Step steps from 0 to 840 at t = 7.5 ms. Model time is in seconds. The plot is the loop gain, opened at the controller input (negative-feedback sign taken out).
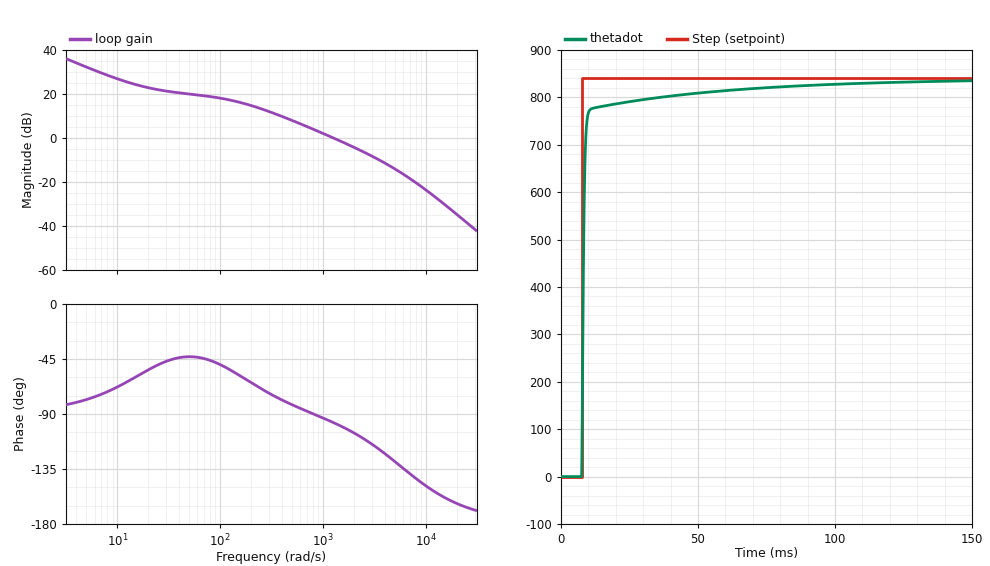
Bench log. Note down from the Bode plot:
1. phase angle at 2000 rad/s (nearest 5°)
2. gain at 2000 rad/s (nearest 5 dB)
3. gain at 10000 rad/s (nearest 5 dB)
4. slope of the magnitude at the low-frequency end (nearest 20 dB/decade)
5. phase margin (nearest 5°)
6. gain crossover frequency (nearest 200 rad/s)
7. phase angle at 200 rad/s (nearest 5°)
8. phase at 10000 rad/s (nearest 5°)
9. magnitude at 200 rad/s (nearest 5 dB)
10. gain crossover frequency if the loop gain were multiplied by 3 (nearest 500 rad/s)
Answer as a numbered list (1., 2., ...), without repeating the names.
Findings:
1. -105°
2. -5 dB
3. -25 dB
4. -20 dB/decade
5. 85°
6. 1200 rad/s
7. -65°
8. -150°
9. 15 dB
10. 3500 rad/s
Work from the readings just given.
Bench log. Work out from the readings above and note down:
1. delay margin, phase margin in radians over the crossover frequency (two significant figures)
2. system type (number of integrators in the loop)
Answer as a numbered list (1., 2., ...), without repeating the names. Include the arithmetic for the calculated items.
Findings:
1. 85 × π / 180 / 1200 = 0.0012 s
2. 1
